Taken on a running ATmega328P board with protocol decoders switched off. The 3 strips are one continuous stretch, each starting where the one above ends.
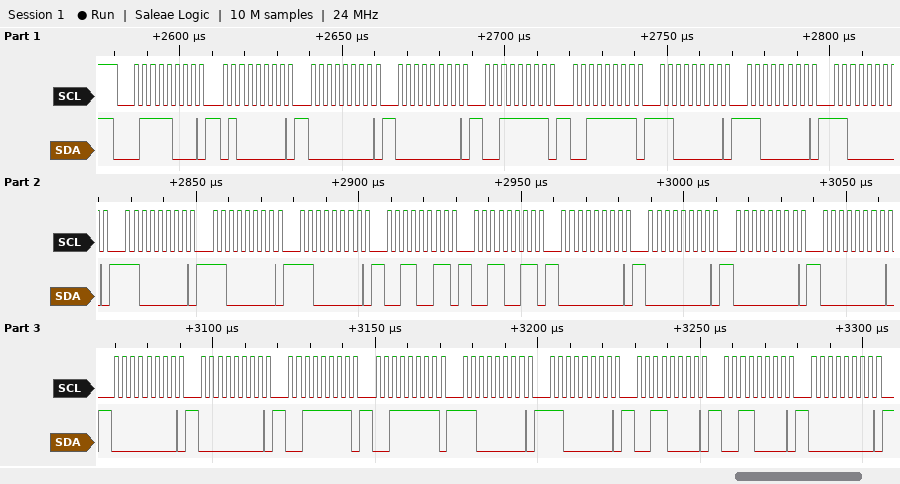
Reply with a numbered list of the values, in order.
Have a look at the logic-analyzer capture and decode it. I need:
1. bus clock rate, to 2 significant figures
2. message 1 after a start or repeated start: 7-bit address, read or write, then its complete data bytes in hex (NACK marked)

1. 400 kHz
2. 0x3C write: 40 00 00 3F 3F C0 C0 C0 C0 C0 C0 33 33 00 00 00 00 00 00 3F 3F C0 C0 30 30 00
